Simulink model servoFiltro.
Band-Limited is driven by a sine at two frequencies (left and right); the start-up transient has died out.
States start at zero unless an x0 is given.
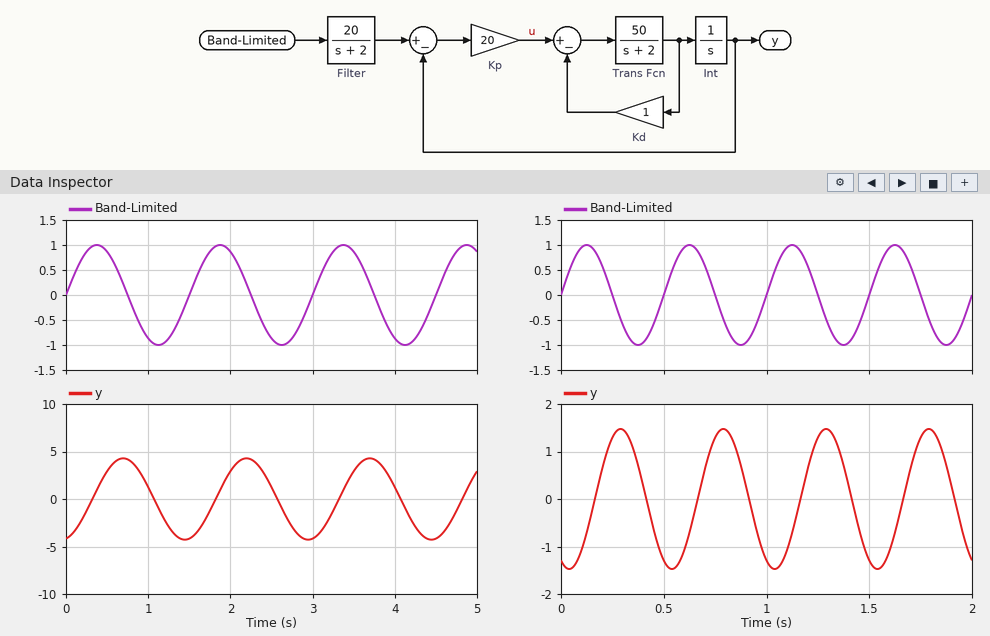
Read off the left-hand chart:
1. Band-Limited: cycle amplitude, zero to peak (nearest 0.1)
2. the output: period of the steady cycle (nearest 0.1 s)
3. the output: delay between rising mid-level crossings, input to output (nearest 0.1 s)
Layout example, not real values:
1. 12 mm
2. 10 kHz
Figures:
1. 1.0
2. 1.5 s
3. 0.3 s
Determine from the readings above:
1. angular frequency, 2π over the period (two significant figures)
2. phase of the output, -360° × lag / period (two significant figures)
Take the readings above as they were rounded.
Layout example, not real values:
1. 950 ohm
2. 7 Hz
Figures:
1. 4.2 rad/s
2. -72°
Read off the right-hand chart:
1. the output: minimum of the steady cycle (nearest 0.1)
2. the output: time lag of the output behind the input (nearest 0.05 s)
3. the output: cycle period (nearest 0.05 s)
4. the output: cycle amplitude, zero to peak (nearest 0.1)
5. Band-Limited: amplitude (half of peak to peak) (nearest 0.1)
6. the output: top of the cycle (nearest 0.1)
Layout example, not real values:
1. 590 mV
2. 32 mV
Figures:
1. -1.5
2. 0.15 s
3. 0.50 s
4. 1.5
5. 1.0
6. 1.5
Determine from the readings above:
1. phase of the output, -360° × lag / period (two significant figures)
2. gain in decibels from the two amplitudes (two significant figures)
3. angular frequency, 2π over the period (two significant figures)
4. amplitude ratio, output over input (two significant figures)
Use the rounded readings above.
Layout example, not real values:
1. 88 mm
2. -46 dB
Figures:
1. -110°
2. 3.5 dB
3. 13 rad/s
4. 1.5
